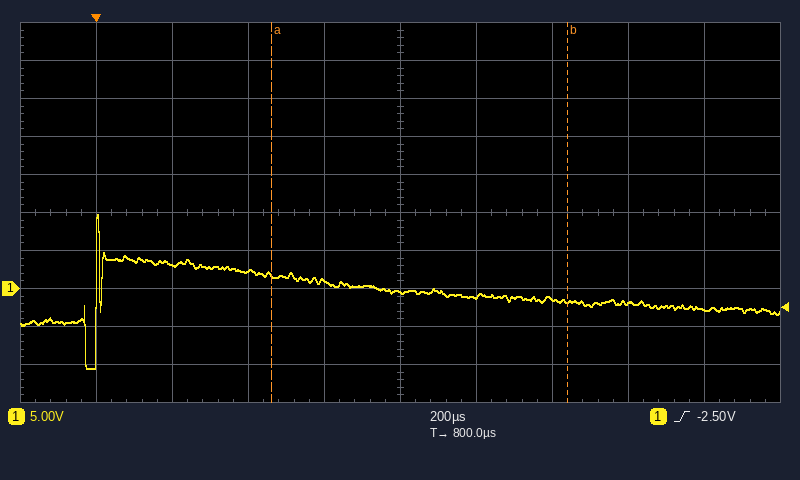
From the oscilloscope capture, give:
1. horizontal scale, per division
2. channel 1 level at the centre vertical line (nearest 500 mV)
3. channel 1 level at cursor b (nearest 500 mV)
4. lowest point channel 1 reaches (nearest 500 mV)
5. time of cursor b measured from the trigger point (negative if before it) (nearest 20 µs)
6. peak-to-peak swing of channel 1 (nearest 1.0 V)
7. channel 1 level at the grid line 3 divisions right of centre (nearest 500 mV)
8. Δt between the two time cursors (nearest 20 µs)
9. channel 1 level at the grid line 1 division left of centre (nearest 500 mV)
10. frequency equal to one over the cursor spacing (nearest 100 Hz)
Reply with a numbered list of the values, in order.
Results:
1. 200 µs
2. -500 mV
3. -1.5 V
4. -10.5 V
5. +1.24 ms
6. 20.0 V
7. -2.0 V
8. 780 µs
9. 1.0 V
10. 1.3 kHz
